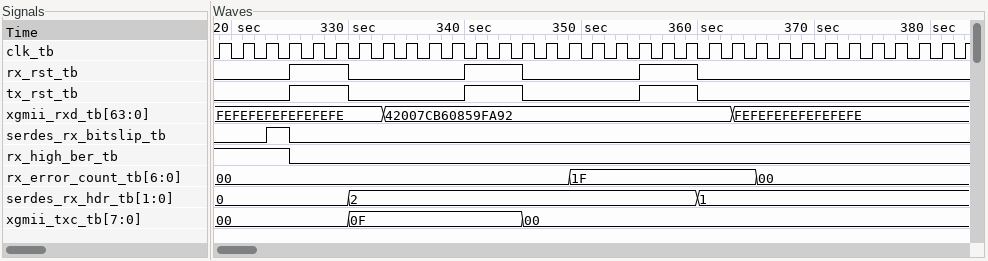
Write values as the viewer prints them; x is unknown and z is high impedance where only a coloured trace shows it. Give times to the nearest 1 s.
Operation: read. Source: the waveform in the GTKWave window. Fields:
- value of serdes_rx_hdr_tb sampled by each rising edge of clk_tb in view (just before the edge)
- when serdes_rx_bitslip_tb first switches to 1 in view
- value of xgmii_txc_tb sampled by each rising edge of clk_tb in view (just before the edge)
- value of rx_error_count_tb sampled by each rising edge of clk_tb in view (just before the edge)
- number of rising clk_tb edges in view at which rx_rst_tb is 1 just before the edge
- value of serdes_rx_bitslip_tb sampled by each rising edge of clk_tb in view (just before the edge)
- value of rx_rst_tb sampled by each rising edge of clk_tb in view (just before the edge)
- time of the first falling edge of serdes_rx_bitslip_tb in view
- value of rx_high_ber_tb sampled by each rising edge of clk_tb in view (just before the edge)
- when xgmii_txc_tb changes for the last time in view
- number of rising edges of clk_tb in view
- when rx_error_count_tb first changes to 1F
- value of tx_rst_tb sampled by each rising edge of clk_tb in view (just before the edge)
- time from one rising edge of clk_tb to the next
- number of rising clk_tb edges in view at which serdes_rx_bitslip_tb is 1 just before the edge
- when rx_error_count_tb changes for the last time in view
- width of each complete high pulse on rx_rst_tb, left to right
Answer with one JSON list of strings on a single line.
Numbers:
["0, 0, 0, 0, 0, 0, 2, 2, 2, 2, 2, 2, 2, 2, 2, 2, 2, 2, 2, 2, 2, 1, 1, 1, 1, 1, 1, 1, 1, 1, 1, 1, 1", "323 s", "00, 00, 00, 00, 00, 00, 0F, 0F, 0F, 0F, 0F, 0F, 0F, 0F, 00, 00, 00, 00, 00, 00, 00, 00, 00, 00, 00, 00, 00, 00, 00, 00, 00, 00, 00", "00, 00, 00, 00, 00, 00, 00, 00, 00, 00, 00, 00, 00, 00, 00, 00, 1F, 1F, 1F, 1F, 1F, 1F, 1F, 1F, 00, 00, 00, 00, 00, 00, 00, 00, 00", "7", "0 0 0 1 0 0 0 0 0 0 0 0 0 0 0 0 0 0 0 0 0 0 0 0 0 0 0 0 0 0 0 0 0", "0 0 0 0 1 1 0 0 0 0 0 1 1 1 0 0 0 0 0 1 1 0 0 0 0 0 0 0 0 0 0 0 0", "325 s", "1 1 1 1 0 0 0 0 0 0 0 0 0 0 0 0 0 0 0 0 0 0 0 0 0 0 0 0 0 0 0 0 0", "345 s", "33", "349 s", "0 0 0 0 1 1 0 0 0 0 0 1 1 1 0 0 0 0 0 1 1 0 0 0 0 0 0 0 0 0 0 0 0", "2 s", "1", "365 s", "5 s, 5 s, 5 s"]
